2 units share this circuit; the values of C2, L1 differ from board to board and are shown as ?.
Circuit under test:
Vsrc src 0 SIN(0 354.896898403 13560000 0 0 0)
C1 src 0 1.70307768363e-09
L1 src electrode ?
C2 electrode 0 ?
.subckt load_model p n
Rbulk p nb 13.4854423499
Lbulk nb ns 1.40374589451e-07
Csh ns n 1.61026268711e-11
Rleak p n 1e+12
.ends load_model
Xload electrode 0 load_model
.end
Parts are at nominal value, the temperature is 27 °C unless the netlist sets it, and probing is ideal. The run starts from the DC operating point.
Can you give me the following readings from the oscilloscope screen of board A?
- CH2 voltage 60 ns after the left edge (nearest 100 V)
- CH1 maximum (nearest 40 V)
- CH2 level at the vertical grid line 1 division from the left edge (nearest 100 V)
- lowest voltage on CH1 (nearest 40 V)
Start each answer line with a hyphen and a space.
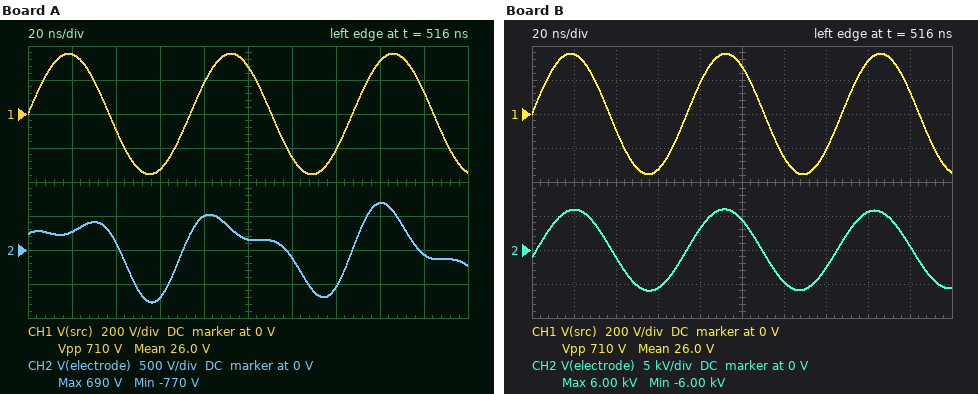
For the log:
- -700 V
- 360 V
- 300 V
- -360 V
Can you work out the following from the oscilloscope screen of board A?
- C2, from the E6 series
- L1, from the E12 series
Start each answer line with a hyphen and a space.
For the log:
- 1.5 nF
- 27 nH
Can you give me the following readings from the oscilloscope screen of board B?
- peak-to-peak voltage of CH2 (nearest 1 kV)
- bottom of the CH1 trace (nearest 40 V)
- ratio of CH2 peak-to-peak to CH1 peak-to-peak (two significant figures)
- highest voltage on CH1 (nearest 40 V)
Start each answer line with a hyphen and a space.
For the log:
- 12 kV
- -360 V
- 17
- 360 V
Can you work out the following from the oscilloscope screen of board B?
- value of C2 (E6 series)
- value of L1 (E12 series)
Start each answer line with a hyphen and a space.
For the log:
- 1 nF
- 120 nH
